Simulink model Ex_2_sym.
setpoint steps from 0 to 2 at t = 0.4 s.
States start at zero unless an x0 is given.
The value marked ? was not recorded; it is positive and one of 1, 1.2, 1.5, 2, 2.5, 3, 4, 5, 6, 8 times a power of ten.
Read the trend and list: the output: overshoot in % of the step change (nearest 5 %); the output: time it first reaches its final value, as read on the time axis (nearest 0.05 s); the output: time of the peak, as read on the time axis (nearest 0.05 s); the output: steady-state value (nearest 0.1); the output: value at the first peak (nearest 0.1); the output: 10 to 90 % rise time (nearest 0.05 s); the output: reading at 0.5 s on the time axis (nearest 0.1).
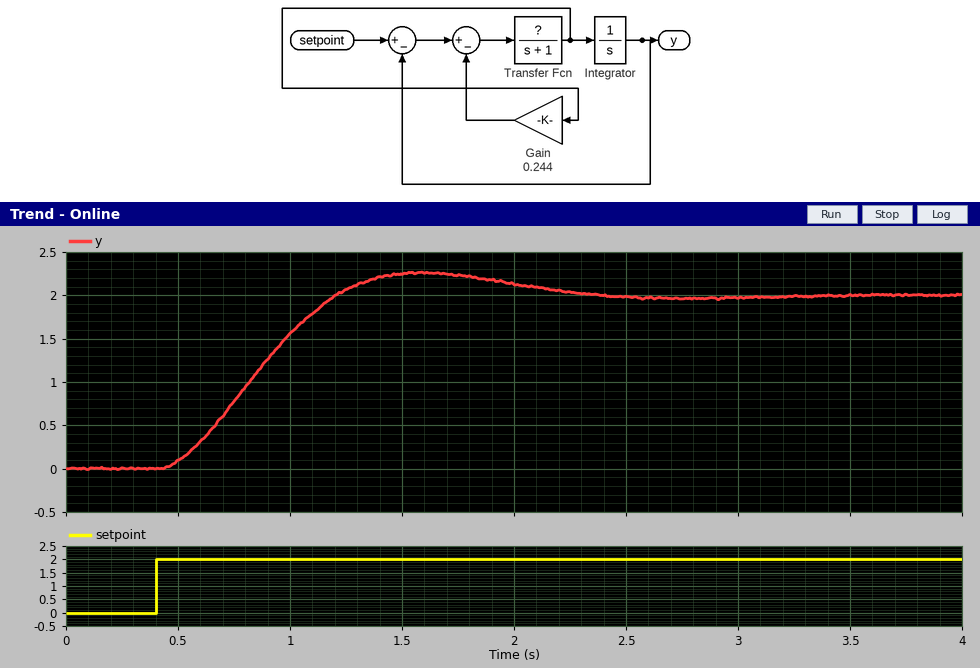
15 %
1.20 s
1.60 s
2.0
2.3
0.55 s
0.1
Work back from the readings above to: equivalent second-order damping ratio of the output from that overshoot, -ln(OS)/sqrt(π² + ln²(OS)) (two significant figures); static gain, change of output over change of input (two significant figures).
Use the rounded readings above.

0.52
1.0
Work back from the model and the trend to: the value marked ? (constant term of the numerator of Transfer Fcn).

10
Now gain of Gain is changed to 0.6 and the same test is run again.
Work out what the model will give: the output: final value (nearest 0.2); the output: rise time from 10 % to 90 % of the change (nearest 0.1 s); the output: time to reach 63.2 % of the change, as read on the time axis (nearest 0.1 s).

2.0
1.2 s
1.1 s
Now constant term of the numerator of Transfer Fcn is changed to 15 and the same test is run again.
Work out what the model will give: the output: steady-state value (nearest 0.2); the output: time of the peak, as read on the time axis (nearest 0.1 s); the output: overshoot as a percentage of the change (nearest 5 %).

2.0
1.4 s
10 %
